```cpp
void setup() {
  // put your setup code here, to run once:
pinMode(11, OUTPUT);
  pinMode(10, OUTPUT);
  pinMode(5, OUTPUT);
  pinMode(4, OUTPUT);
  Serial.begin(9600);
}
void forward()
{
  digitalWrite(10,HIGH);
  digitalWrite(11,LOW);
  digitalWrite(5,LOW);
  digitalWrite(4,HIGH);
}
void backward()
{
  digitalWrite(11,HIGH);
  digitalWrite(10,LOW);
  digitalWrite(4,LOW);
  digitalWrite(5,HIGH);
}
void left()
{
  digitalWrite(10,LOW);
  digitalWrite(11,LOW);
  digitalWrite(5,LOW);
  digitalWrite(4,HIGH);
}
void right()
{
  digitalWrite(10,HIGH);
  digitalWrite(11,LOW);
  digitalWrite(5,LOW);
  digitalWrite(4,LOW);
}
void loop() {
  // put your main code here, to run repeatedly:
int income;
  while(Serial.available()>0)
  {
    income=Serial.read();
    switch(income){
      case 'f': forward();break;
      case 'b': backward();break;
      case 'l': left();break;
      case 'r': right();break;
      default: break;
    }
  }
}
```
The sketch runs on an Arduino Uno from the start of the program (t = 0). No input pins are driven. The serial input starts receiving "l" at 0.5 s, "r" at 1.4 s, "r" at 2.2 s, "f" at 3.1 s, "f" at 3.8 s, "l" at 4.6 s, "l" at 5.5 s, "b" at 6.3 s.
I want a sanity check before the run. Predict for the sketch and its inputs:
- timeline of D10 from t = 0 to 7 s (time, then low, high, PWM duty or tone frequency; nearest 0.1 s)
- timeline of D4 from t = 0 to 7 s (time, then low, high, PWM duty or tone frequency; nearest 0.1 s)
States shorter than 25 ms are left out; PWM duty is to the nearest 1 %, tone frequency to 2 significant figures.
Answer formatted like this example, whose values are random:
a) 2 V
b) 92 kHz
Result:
a) 0 s low; 1.4 s high; 4.6 s low
b) 0 s low; 0.5 s high; 1.4 s low; 3.1 s high; 6.3 s low
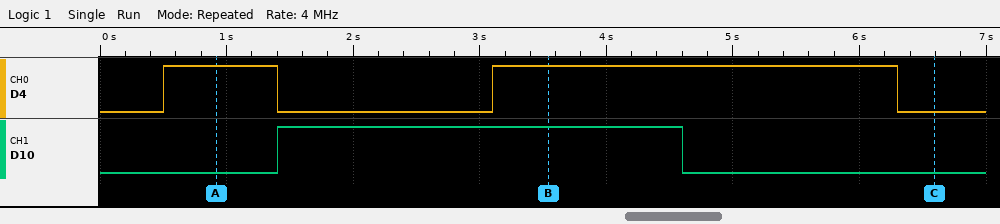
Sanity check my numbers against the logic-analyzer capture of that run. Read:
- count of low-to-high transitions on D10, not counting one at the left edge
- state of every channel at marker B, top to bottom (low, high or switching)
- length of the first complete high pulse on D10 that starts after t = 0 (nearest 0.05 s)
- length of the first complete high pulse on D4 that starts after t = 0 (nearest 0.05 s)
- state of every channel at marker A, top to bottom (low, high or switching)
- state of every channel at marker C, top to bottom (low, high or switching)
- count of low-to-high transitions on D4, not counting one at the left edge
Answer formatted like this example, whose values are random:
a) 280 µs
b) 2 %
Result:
a) 1
b) D4 high, D10 high
c) 3.20 s
d) 0.90 s
e) D4 high, D10 low
f) D4 low, D10 low
g) 2
